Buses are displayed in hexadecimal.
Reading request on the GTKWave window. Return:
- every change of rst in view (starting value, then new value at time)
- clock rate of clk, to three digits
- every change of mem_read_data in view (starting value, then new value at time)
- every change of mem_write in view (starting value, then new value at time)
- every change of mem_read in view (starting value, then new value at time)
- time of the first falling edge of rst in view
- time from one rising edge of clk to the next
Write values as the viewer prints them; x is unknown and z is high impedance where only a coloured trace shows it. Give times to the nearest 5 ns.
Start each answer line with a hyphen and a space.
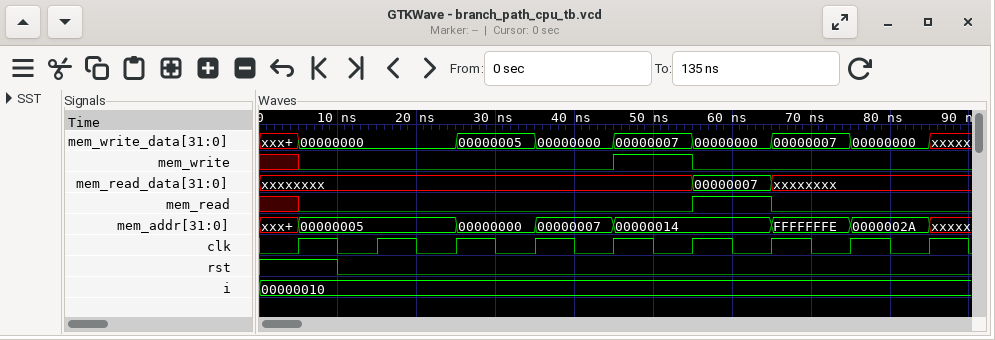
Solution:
- 1, 0 at 10 ns
- 100 MHz
- xxxxxxxx, 00000007 at 55 ns, xxxxxxxx at 65 ns
- x, 0 at 5 ns, 1 at 45 ns, 0 at 55 ns
- x, 0 at 5 ns, 1 at 55 ns, 0 at 65 ns
- 10 ns
- 10 ns
